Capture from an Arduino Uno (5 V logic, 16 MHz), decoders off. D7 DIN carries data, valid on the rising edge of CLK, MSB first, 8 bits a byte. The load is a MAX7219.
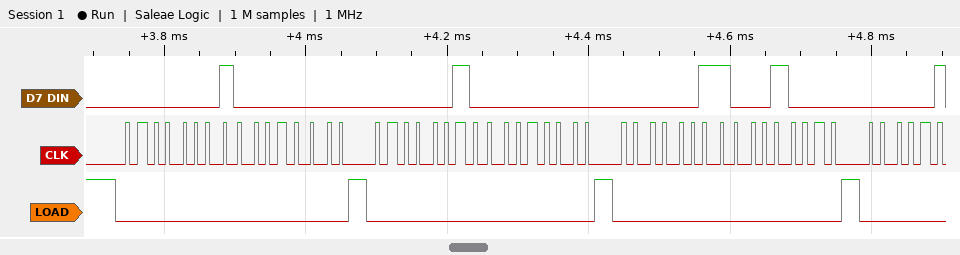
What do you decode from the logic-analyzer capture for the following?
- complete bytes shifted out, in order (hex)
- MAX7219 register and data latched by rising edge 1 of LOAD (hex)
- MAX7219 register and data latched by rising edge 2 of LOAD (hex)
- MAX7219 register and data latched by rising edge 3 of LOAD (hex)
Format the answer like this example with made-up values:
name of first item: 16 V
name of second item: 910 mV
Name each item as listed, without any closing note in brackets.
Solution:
complete bytes shifted out, in order: 01 00 02 00 03 10
MAX7219 register and data latched by rising edge 1 of LOAD: register 0x1, data 0x00
MAX7219 register and data latched by rising edge 2 of LOAD: register 0x2, data 0x00
MAX7219 register and data latched by rising edge 3 of LOAD: register 0x3, data 0x10
